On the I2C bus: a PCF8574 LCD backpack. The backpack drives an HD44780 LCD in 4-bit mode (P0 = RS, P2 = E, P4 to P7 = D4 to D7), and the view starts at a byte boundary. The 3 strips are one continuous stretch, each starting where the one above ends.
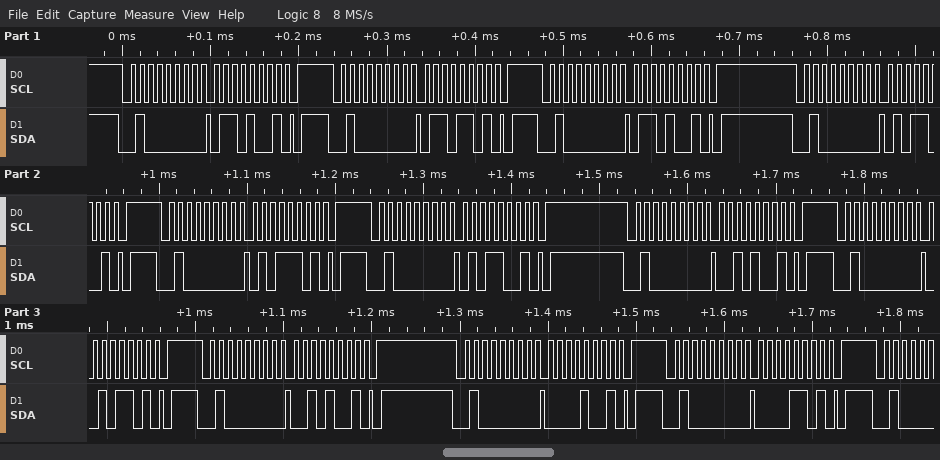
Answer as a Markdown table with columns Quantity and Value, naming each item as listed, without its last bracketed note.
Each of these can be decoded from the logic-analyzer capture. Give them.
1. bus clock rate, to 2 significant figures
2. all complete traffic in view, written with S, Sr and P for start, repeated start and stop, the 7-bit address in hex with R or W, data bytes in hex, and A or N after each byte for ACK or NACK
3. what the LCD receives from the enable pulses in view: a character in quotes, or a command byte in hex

| Quantity | Value |
|---|---|
| bus clock rate, to 2 significant figures | 100 kHz |
| all complete traffic in view, written with S, Sr and P for start, repeated start and stop, the 7-bit address in hex with R or W, data bytes in hex, and A or N after each byte for ACK or NACK | S 20W A 69 A P S 20W A 6D A P S 20W A 69 A P S 20W A 59 A P S 20W A 5D A P S 20W A 59 A P S 20W A 29 A P S 20W A 2D A P S 20W A 29 A P S 20W A 09 A P S 20W A 0D A P |
| what the LCD receives from the enable pulses in view: a character in quotes, or a command byte in hex | 'e' |
